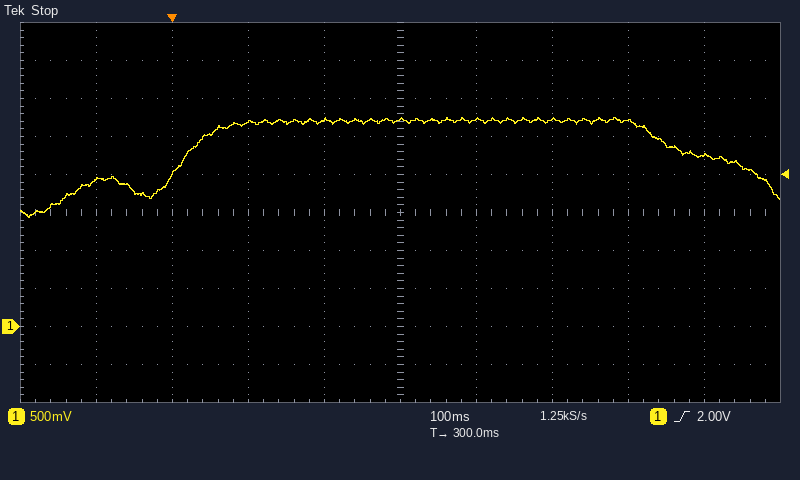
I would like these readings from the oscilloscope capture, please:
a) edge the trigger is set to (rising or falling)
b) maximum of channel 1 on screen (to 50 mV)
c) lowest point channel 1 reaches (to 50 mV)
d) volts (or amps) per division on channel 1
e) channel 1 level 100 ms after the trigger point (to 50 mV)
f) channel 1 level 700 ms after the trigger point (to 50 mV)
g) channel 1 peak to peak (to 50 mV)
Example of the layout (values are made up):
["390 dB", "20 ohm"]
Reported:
["rising", "2.75 V", "1.45 V", "500 mV", "2.70 V", "2.25 V", "1.30 V"]
